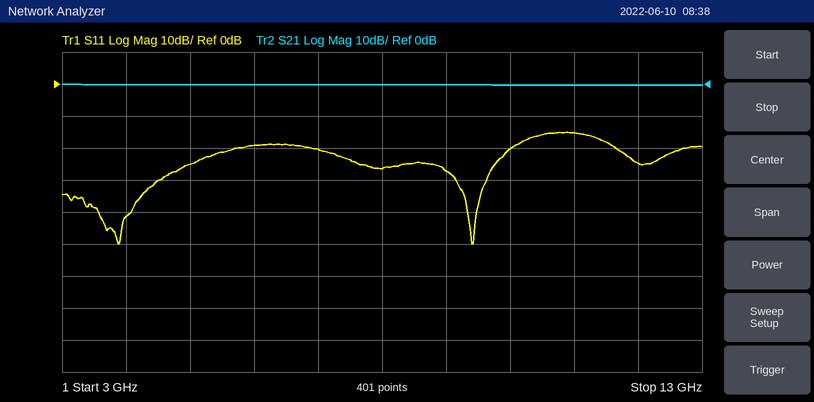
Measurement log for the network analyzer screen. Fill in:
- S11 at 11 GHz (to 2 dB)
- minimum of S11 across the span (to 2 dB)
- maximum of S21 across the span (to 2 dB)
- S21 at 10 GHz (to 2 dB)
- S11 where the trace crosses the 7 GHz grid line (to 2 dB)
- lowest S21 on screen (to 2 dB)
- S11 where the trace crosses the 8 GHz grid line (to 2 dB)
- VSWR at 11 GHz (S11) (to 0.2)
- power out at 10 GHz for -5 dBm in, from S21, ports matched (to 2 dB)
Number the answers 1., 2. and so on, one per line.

1. -16 dB
2. -50 dB
3. 0 dB
4. 0 dB
5. -20 dB
6. 0 dB
7. -26 dB
8. 1.4
9. -6 dBm
